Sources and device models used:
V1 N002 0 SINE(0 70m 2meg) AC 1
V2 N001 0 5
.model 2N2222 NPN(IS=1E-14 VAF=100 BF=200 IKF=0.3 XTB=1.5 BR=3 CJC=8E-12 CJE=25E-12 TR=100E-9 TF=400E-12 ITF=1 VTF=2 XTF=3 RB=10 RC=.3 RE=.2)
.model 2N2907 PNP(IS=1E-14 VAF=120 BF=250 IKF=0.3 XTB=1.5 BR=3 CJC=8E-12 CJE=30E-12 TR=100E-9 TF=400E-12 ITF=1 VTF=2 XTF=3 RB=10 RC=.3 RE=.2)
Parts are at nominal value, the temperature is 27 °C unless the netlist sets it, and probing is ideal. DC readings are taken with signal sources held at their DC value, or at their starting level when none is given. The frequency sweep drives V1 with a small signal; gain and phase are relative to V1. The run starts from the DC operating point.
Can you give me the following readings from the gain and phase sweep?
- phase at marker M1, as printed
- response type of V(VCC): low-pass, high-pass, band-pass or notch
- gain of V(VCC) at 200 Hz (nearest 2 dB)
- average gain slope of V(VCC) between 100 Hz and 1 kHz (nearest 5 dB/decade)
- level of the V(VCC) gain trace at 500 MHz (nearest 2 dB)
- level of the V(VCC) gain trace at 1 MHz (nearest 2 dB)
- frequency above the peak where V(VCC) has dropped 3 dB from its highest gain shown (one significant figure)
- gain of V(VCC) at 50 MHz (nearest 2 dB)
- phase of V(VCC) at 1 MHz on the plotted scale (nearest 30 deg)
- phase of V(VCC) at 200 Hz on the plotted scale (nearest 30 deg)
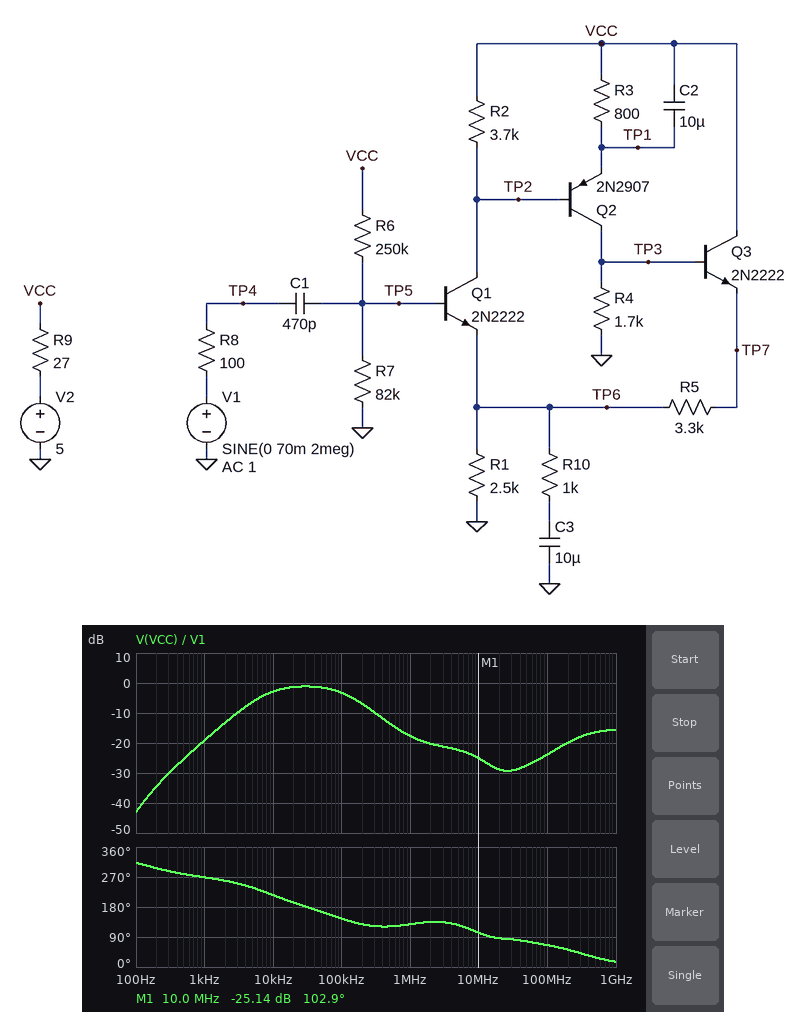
102.9 deg
band-pass
-34 dB
25 dB/decade
-16 dB
-18 dB
100 kHz
-28 dB
120 deg
300 deg
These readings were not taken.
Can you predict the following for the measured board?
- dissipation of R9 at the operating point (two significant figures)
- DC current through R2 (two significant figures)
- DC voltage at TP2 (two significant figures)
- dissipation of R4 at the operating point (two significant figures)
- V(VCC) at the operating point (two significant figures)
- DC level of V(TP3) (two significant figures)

6.0 µW
220 µA
4.2 V
96 µW
5.0 V
400 mV
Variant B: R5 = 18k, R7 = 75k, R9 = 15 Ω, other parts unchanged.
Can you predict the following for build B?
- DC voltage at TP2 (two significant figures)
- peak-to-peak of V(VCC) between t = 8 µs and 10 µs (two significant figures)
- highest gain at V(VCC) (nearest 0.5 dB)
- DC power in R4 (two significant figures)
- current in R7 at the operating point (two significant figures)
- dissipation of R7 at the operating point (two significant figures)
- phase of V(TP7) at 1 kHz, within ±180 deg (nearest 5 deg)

4.3 V
11 mV
-10.5 dB
33 µW
15 µA
16 µW
90 deg
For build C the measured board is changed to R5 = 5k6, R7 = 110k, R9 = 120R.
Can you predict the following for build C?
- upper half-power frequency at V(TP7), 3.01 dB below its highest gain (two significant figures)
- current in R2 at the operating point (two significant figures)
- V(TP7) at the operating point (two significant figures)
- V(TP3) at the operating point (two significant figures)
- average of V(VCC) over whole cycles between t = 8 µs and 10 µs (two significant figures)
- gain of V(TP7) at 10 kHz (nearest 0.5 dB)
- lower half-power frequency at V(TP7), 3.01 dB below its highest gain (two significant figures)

5.2 MHz
300 µA
760 mV
990 mV
4.9 V
-2.0 dB
42 kHz
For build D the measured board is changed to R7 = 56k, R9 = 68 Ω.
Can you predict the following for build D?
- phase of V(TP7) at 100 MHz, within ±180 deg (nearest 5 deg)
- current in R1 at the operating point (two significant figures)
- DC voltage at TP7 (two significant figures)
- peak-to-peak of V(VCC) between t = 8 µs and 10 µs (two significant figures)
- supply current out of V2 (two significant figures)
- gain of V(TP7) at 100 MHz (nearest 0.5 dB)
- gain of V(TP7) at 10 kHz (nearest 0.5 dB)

40 deg
120 µA
290 mV
8.7 mV
130 µA
-20.0 dB
-5.5 dB
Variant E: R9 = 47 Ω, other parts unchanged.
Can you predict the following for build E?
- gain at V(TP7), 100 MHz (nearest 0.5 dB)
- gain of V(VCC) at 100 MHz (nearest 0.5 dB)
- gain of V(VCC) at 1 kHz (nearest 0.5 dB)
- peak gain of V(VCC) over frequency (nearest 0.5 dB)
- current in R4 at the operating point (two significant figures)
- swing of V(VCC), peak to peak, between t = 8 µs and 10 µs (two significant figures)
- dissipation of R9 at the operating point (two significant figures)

-15.0 dB
-19.5 dB
-15.5 dB
3.5 dB
230 µA
23 mV
10 µW
